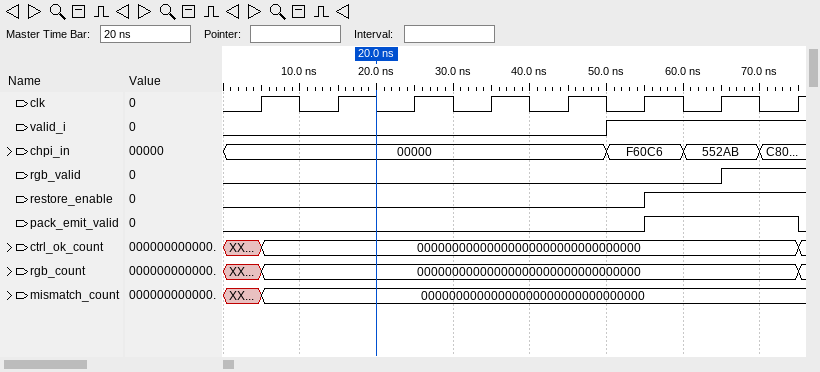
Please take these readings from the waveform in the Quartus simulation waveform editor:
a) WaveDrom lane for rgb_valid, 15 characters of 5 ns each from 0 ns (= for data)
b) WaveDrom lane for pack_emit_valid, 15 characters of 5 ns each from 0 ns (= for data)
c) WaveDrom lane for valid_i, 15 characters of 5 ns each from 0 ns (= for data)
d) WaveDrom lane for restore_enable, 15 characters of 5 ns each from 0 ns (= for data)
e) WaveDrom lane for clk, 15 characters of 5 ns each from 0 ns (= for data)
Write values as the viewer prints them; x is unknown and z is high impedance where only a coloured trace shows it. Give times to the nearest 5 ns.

{name: 'rgb_valid', wave: '0............1.'}
{name: 'pack_emit_valid', wave: '0..........1...'}
{name: 'valid_i', wave: '0.........1....'}
{name: 'restore_enable', wave: '0..........1...'}
{name: 'clk', wave: '010101010101010'}
